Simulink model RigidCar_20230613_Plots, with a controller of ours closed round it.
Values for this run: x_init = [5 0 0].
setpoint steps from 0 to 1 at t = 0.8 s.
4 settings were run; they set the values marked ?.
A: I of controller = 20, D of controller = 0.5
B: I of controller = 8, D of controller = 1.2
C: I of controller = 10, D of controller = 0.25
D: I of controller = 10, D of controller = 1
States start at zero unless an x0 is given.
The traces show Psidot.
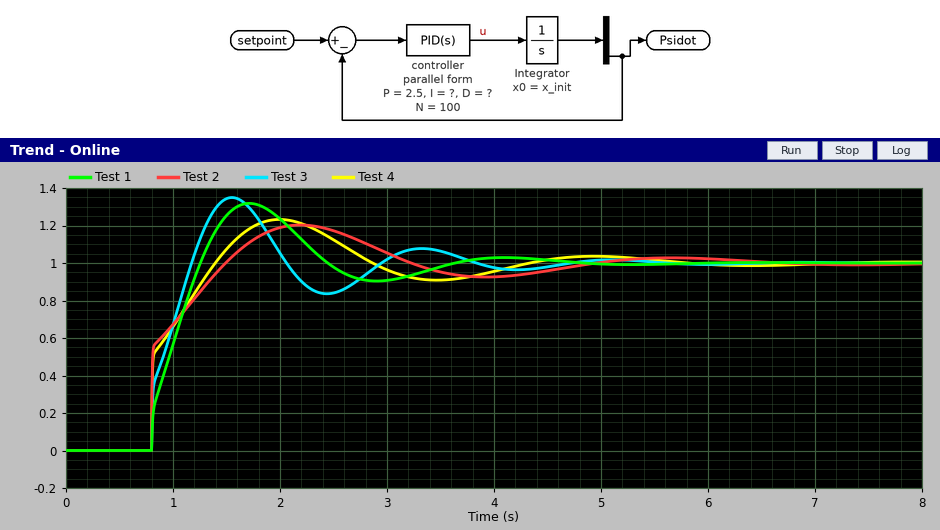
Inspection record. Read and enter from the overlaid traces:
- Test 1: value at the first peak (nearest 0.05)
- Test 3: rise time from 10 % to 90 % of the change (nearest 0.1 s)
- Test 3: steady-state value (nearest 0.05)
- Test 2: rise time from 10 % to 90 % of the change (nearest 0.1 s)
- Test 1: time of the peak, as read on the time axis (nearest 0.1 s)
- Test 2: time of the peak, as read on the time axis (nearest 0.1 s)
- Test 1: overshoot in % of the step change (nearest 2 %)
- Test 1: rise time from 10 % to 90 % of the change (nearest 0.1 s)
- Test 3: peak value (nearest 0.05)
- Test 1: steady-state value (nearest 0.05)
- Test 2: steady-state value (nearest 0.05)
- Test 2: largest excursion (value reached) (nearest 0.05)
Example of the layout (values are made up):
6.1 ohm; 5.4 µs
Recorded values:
1.30; 0.3 s; 1.00; 0.5 s; 1.7 s; 2.2 s; 32 %; 0.4 s; 1.35; 1.00; 1.00; 1.20
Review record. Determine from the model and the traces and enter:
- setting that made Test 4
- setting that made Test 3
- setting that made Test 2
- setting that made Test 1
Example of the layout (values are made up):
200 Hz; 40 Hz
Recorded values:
D; A; B; C
